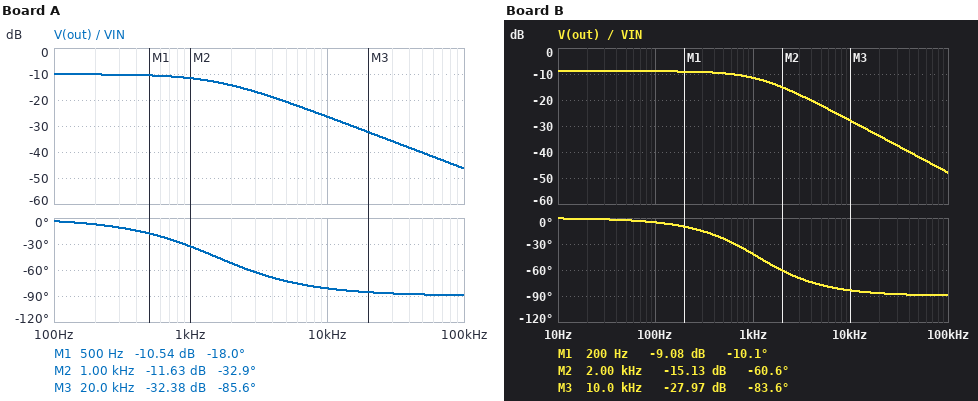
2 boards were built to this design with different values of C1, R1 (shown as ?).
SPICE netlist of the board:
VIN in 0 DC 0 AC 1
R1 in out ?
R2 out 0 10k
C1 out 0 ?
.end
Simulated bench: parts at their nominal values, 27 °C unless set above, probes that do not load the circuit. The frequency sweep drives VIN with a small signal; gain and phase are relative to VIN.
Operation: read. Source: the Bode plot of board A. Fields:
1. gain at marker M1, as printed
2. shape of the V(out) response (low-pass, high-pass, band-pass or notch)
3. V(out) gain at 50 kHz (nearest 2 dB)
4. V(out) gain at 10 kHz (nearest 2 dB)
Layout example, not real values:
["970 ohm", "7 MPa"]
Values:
["-10.54 dB", "low-pass", "-40 dB", "-26 dB"]
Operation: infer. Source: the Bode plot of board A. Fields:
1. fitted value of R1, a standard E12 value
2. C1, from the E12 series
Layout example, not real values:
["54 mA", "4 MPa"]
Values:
["22 kΩ", "15 nF"]
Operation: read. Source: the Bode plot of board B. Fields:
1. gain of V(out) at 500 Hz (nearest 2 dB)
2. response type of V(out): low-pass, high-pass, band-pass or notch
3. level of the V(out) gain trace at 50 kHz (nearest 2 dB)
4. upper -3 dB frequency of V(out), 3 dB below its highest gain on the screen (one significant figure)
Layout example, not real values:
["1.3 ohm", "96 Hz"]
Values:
["-10 dB", "low-pass", "-42 dB", "1 kHz"]
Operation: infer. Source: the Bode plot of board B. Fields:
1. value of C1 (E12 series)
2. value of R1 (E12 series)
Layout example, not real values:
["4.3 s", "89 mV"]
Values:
["22 nF", "18 kΩ"]
